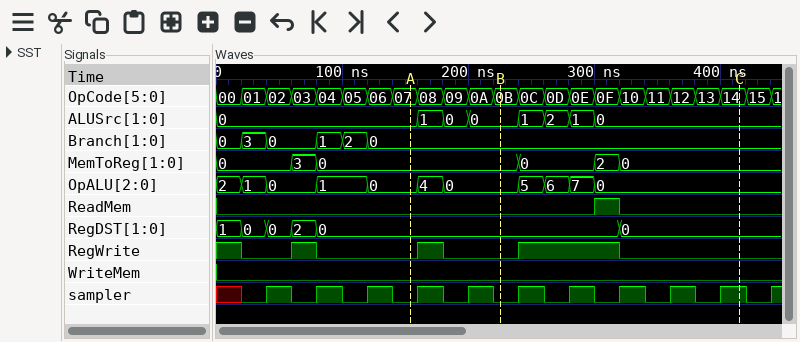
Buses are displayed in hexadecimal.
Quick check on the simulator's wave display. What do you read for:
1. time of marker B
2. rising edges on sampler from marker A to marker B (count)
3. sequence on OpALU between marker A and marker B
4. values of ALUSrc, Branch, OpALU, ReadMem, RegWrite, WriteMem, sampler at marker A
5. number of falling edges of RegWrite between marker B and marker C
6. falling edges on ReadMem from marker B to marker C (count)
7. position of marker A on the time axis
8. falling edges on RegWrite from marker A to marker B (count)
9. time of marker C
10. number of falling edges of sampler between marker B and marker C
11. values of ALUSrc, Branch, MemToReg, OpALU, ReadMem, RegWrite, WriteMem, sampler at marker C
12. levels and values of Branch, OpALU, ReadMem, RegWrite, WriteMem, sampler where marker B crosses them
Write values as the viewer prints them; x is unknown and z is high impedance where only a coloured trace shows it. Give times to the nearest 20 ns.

220 ns
2
0, 4, 0
ALUSrc=0, Branch=0, OpALU=0, ReadMem=0, RegWrite=0, WriteMem=0, sampler=0
1
1
160 ns
1
420 ns
4
ALUSrc=0, Branch=0, MemToReg=0, OpALU=0, ReadMem=0, RegWrite=0, WriteMem=0, sampler=1
Branch=0, OpALU=0, ReadMem=0, RegWrite=0, WriteMem=0, sampler=0
